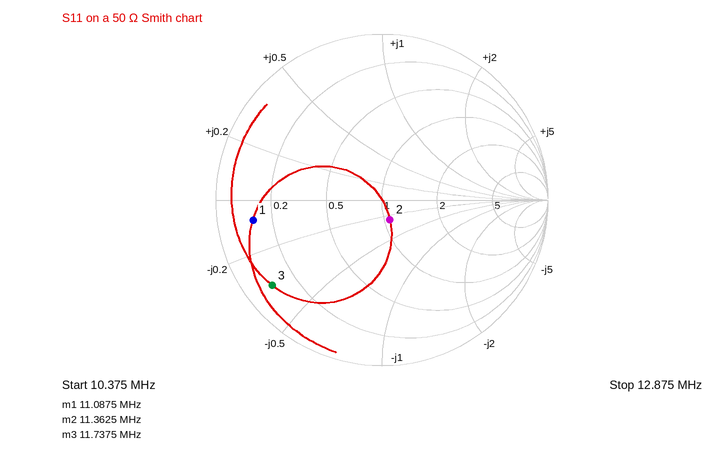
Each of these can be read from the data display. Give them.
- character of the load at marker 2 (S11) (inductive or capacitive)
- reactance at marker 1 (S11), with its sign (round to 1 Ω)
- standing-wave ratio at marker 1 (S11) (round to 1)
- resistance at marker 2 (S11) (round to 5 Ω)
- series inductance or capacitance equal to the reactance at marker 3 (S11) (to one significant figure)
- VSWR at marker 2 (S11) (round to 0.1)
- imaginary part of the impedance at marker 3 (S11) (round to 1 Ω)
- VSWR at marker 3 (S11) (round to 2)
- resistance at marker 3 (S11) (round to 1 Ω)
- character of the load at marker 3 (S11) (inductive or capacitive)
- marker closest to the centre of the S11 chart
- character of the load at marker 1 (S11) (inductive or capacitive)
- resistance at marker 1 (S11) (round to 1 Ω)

capacitive
-4 Ω
8
55 Ω
800 pF
1.3
-17 Ω
12
5 Ω
capacitive
marker 2
capacitive
6 Ω
